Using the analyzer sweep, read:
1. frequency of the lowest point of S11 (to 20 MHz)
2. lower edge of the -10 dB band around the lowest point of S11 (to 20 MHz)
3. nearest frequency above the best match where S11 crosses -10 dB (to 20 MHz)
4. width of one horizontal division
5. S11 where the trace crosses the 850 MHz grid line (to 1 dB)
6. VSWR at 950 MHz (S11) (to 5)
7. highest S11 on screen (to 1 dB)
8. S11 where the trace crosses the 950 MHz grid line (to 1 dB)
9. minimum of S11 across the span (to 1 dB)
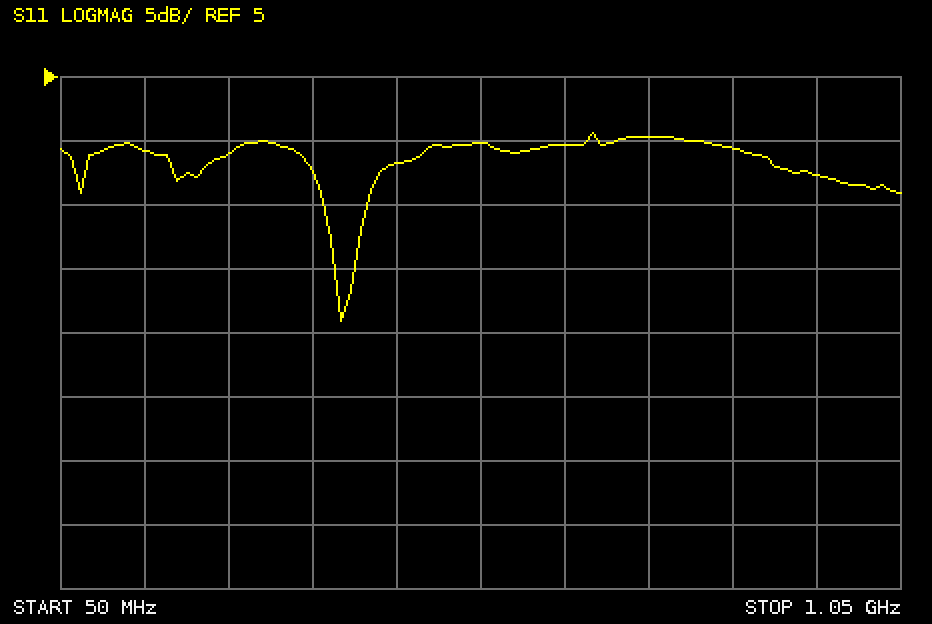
380 MHz
380 MHz
400 MHz
100 MHz
-1 dB
5
1 dB
-3 dB
-14 dB
